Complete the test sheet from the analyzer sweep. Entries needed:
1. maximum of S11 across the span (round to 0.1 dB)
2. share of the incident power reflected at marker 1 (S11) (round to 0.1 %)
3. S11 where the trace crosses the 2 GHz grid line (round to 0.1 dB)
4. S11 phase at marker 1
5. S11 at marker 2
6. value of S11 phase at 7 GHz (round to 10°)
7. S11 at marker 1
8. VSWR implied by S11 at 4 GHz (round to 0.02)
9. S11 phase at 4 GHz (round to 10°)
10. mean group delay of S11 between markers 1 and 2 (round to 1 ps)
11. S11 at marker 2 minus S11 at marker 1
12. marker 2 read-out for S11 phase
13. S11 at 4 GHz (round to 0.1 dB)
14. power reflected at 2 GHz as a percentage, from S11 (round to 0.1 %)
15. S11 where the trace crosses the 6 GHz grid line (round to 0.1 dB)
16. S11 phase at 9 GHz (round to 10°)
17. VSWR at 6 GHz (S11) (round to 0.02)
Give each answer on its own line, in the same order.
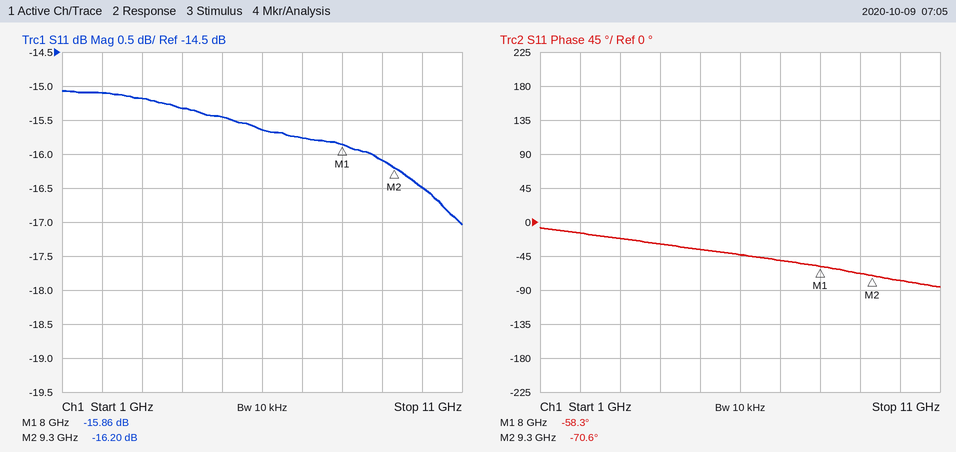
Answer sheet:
-15.1 dB
2.6 %
-15.1 dB
-58.3°
-16.20 dB
-50°
-15.86 dB
1.42
-30°
26 ps
-0.34 dB
-70.6°
-15.3 dB
3.1 %
-15.6 dB
-70°
1.40
